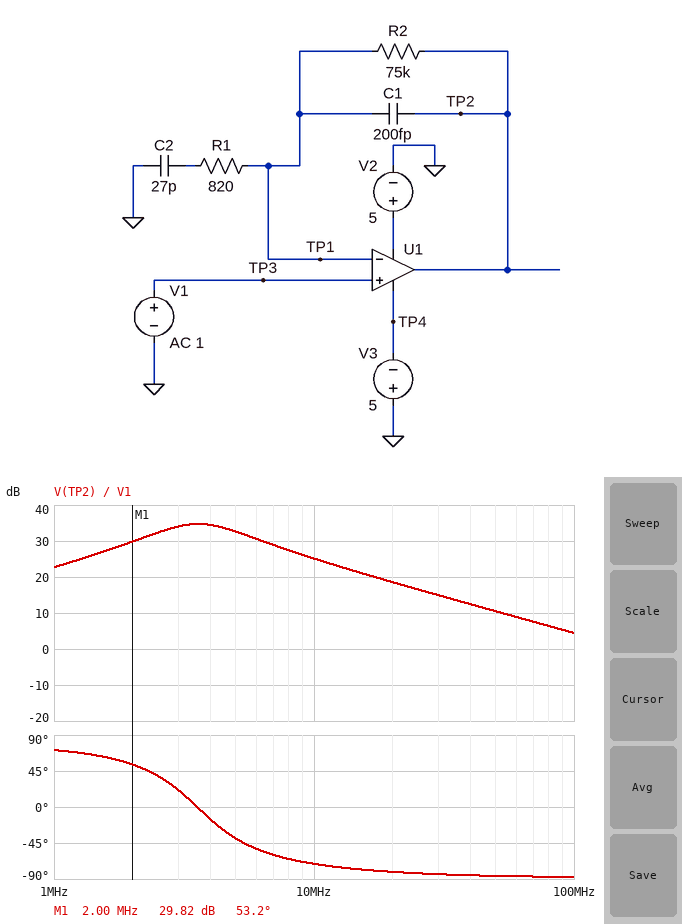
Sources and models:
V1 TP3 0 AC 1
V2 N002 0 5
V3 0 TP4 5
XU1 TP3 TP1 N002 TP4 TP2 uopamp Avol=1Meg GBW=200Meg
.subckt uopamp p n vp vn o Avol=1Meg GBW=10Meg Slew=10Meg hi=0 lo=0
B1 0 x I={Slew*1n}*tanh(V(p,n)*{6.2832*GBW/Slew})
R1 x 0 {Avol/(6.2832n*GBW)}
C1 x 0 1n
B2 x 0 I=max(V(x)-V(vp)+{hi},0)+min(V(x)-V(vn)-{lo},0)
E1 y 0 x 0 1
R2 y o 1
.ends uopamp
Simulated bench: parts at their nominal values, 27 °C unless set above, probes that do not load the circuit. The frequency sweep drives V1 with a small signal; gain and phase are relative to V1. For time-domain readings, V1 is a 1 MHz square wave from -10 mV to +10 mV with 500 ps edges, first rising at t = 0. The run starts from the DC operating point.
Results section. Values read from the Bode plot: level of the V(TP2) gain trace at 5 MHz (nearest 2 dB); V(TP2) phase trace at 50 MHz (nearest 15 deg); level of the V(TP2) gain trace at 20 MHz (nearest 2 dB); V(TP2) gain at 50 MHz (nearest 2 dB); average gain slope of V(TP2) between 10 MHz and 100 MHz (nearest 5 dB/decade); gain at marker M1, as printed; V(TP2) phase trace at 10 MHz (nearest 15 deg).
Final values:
32 dB
-90 deg
18 dB
10 dB
-20 dB/decade
29.82 dB
-75 deg
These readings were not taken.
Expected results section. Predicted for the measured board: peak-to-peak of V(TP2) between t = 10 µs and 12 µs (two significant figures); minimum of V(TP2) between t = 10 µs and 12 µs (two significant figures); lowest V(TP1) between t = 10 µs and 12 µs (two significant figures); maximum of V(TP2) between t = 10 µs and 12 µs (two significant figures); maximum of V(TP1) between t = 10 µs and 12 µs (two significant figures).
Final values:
1.0 V
-510 mV
-16 mV
510 mV
16 mV
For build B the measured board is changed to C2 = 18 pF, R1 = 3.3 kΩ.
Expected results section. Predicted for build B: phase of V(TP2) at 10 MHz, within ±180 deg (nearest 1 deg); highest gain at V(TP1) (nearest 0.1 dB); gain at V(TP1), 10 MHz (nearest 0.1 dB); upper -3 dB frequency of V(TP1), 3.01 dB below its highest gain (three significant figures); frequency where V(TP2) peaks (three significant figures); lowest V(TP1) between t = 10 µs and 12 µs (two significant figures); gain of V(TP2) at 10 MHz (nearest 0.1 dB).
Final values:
-55 deg
0.8 dB
-3.9 dB
6.86 MHz
3.56 MHz
-12 mV
20.6 dB
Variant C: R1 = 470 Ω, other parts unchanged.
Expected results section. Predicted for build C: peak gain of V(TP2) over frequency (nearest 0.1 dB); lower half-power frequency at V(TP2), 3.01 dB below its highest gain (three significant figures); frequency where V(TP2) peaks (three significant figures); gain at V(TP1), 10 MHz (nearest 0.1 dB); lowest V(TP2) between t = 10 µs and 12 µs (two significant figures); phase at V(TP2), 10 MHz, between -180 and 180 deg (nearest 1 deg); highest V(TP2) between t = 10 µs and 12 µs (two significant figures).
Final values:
37.2 dB
2.69 MHz
3.73 MHz
-11.3 dB
-570 mV
-74 deg
570 mV
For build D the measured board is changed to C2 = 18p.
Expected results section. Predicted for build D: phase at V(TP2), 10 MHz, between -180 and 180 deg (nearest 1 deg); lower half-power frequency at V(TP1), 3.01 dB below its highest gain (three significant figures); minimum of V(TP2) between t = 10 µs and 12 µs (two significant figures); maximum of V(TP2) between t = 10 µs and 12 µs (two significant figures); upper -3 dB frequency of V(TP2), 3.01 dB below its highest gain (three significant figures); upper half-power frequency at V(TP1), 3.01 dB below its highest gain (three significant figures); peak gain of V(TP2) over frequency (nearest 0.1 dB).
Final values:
-66 deg
925 kHz
-410 mV
410 mV
6.60 MHz
5.57 MHz
33.1 dB
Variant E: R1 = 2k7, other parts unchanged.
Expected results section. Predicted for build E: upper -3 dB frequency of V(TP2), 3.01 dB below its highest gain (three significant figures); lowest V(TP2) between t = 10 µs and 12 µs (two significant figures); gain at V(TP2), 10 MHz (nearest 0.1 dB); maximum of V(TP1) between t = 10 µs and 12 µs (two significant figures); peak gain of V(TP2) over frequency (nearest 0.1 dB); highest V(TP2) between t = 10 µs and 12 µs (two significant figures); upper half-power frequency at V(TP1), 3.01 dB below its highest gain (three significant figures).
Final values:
6.53 MHz
-320 mV
21.4 dB
12 mV
27.6 dB
320 mV
5.71 MHz
